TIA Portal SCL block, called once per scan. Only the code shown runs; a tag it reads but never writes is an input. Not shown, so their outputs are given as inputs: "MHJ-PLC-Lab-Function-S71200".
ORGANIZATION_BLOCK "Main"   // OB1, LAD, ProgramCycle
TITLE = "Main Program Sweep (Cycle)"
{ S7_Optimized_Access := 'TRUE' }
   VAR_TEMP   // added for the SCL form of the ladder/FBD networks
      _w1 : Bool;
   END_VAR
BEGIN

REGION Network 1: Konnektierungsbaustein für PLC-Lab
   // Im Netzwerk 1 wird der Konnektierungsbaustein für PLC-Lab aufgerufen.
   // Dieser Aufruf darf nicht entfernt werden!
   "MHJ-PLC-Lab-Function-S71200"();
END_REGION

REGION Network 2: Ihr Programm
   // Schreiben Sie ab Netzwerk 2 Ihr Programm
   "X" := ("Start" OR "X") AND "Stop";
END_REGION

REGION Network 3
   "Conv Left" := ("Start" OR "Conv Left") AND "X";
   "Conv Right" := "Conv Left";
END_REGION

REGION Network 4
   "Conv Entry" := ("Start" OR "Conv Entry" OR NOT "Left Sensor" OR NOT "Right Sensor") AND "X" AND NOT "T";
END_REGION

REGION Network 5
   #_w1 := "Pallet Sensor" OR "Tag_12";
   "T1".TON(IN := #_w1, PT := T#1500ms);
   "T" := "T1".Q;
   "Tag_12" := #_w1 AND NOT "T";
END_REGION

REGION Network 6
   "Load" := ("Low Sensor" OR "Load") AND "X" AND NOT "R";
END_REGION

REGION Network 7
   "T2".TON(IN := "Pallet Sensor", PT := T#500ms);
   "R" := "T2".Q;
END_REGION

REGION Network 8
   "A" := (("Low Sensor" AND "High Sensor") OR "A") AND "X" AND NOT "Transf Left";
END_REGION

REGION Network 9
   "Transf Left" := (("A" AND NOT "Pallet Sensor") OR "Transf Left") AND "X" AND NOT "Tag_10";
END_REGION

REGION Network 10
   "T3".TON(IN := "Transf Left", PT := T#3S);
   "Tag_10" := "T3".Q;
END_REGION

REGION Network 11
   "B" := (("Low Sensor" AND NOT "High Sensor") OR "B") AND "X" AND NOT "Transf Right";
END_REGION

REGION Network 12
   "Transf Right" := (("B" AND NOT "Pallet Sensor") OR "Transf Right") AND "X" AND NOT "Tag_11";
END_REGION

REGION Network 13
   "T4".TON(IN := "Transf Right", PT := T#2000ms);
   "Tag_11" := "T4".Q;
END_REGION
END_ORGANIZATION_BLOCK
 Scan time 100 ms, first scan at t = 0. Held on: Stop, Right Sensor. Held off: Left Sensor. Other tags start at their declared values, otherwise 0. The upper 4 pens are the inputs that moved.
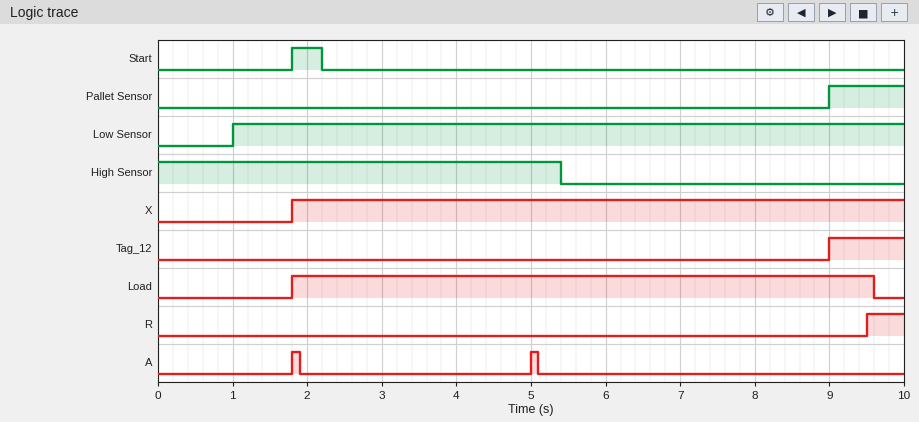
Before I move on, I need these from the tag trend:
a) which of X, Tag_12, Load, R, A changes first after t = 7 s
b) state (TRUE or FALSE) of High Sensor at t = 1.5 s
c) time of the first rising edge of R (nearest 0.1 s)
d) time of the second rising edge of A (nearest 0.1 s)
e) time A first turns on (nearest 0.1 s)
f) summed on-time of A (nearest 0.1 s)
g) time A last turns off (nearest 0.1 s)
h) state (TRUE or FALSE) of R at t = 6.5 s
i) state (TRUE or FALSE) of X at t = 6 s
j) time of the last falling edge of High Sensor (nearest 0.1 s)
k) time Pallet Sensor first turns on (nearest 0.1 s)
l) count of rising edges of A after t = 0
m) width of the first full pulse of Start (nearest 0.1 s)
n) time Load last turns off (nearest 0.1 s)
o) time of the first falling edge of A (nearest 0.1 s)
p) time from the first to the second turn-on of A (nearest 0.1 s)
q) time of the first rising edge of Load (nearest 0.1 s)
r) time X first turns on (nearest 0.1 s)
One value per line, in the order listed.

Tag_12
TRUE
9.5 s
5.0 s
1.8 s
0.2 s
5.1 s
FALSE
TRUE
5.4 s
9.0 s
2
0.4 s
9.6 s
1.9 s
3.2 s
1.8 s
1.8 s
